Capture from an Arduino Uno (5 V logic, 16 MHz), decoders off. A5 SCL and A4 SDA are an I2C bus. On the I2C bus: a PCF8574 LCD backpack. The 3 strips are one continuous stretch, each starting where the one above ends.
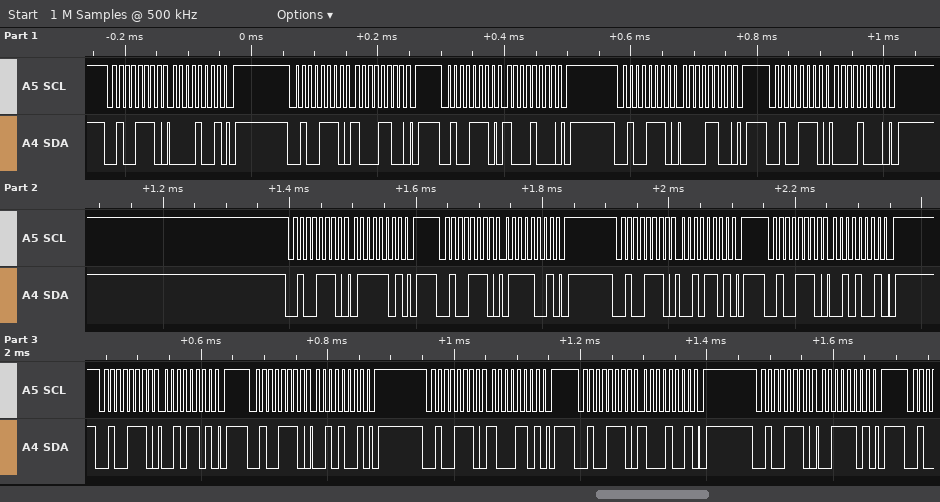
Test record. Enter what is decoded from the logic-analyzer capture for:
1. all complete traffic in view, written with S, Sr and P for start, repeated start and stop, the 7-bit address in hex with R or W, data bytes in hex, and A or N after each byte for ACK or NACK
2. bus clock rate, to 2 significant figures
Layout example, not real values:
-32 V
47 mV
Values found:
S 27W A 09 A P S 27W A 8C A P S 27W A 88 A P S 27W A 0C A P S 27W A 08 A P S 27W A 7D A P S 27W A 79 A P S 27W A 2D A P S 27W A 29 A P S 27W A 2D A P S 27W A 29 A P S 27W A 8D A P S 27W A 89 A P S 27W A 3D A P
100 kHz
